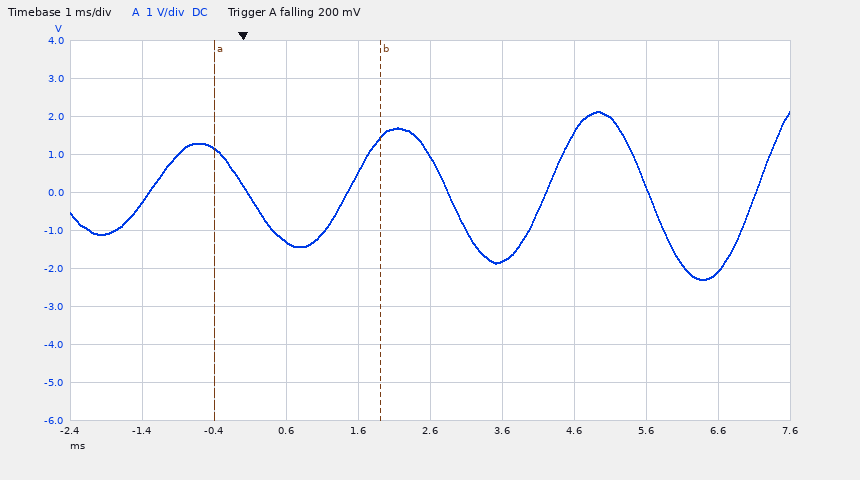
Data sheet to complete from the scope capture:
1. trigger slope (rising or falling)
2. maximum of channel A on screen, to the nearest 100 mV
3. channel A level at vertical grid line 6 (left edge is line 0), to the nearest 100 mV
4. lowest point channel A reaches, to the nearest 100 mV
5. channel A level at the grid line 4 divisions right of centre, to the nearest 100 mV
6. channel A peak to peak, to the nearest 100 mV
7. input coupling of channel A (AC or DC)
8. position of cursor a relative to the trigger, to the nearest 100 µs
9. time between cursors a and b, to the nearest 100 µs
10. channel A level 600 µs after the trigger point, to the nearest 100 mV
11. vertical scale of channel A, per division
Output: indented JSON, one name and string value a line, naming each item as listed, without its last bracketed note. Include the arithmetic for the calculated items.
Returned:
{
  "trigger slope": "falling",
  "maximum of channel A on screen, to the nearest 100 mV": "2.1 V",
  "channel A level at vertical grid line 6 (left edge is line 0), to the nearest 100 mV": "-1.8 V",
  "lowest point channel A reaches, to the nearest 100 mV": "-2.3 V",
  "channel A level at the grid line 4 divisions right of centre, to the nearest 100 mV": "-2.1 V",
  "channel A peak to peak, to the nearest 100 mV": "2.1 V − (-2.3 V) = 4.4 V",
  "input coupling of channel A": "DC",
  "position of cursor a relative to the trigger, to the nearest 100 µs": "-400 µs",
  "time between cursors a and b, to the nearest 100 µs": "2.3 ms",
  "channel A level 600 µs after the trigger point, to the nearest 100 mV": "-1.3 V",
  "vertical scale of channel A, per division": "1 V"
}
